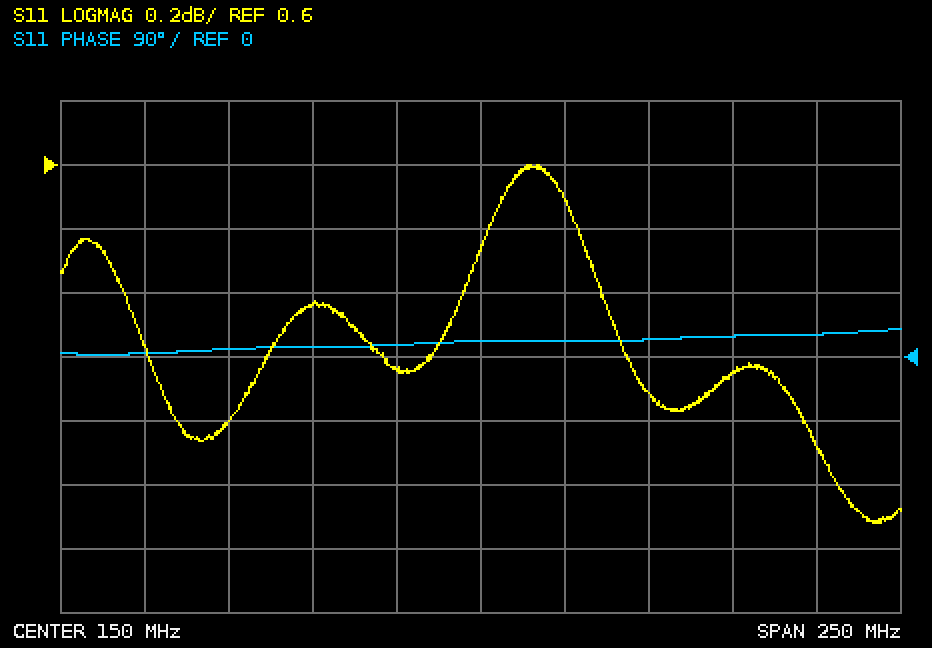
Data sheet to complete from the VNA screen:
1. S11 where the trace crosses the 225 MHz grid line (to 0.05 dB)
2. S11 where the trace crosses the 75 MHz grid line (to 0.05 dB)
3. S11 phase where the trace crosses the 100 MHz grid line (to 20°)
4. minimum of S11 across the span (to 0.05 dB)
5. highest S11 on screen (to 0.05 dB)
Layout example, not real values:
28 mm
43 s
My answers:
-0.05 dB
-0.20 dB
20°
-0.50 dB
0.60 dB
